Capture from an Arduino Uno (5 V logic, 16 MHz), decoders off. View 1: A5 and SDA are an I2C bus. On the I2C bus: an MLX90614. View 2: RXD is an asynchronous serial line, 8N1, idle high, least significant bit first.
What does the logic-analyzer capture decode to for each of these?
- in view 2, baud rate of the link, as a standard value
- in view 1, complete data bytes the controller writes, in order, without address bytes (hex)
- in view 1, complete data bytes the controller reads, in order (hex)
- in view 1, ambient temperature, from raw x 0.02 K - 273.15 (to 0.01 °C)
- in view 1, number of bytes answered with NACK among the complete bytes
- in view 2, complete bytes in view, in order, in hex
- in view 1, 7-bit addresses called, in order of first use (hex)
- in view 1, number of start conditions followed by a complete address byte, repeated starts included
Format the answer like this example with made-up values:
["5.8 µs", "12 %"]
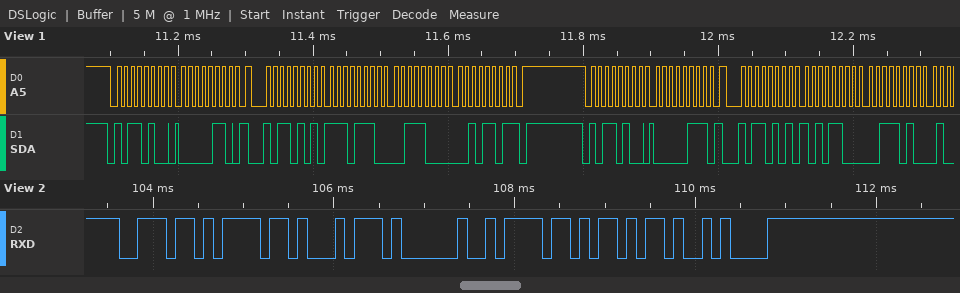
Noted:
["9600 baud", "06 07", "EE 38 2D AC 3A", "18.33 °C", "1", "6E 6F 74 20 6F 6B 0A", "0x5A", "4"]
